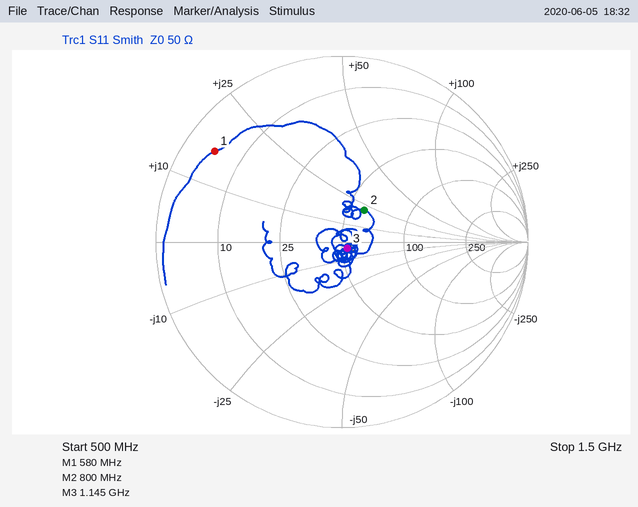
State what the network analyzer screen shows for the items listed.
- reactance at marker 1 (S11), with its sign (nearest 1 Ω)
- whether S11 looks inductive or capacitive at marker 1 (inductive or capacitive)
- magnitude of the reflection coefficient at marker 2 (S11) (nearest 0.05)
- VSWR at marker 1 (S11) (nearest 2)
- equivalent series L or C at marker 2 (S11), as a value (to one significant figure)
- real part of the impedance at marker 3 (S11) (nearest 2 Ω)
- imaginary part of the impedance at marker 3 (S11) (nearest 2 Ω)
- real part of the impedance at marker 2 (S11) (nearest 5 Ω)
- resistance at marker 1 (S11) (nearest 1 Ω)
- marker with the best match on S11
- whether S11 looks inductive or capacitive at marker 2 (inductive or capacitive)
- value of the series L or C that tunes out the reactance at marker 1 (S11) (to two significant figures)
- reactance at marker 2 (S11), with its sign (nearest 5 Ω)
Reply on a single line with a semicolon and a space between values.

+16 Ω; inductive; 0.20; 12; 4 nH; 52 Ω; -4 Ω; 60 Ω; 5 Ω; marker 3; inductive; 17 pF; +20 Ω
